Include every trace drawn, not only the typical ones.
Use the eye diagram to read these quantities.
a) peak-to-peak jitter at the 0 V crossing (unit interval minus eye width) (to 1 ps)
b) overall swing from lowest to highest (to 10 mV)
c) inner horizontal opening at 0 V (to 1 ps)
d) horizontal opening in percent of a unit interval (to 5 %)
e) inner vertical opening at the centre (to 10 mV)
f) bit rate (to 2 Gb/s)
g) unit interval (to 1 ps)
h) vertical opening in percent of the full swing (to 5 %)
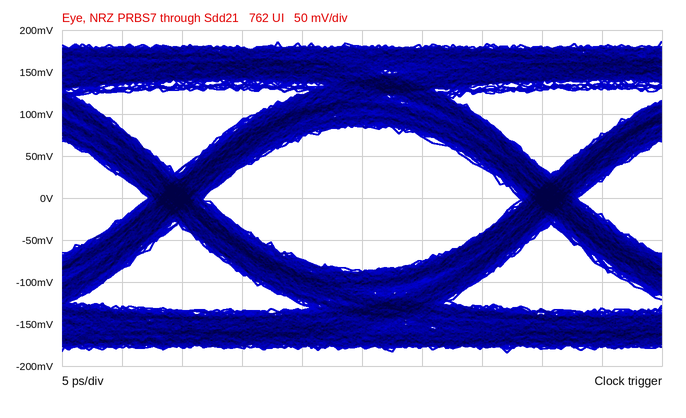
5 ps
370 mV
26 ps
85 %
170 mV
32 Gb/s
31 ps
45 %
